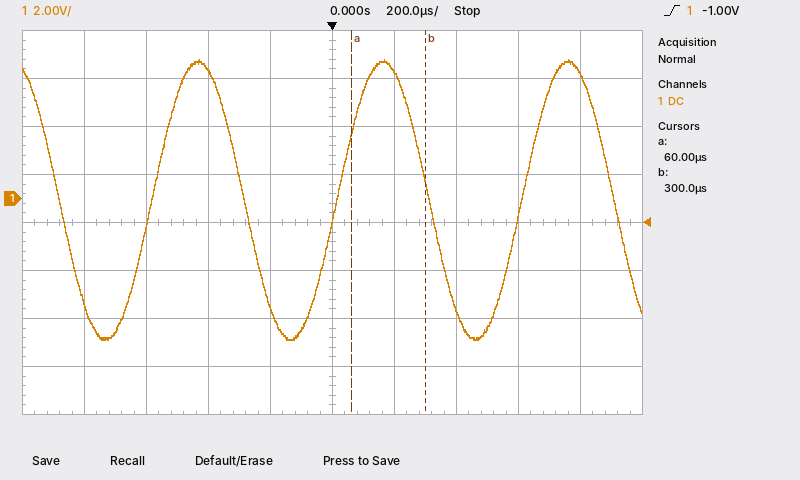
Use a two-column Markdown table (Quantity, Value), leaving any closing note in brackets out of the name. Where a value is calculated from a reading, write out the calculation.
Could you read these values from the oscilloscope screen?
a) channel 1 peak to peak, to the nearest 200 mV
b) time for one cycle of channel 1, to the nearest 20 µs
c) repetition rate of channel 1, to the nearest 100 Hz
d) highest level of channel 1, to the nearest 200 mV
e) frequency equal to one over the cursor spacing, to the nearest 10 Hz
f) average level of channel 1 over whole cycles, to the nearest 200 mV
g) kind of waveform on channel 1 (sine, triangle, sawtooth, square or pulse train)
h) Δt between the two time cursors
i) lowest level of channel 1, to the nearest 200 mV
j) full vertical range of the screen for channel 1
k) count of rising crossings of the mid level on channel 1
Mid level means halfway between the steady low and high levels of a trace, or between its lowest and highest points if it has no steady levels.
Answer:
| Quantity | Value |
|---|---|
| channel 1 peak to peak, to the nearest 200 mV | 5.8 V − (-5.8 V) = 11.6 V |
| time for one cycle of channel 1, to the nearest 20 µs | 600 µs |
| repetition rate of channel 1, to the nearest 100 Hz | 1 / 600 µs ≈ 1.7 kHz |
| highest level of channel 1, to the nearest 200 mV | 5.8 V |
| frequency equal to one over the cursor spacing, to the nearest 10 Hz | 1 / 240 µs ≈ 4.17 kHz |
| average level of channel 1 over whole cycles, to the nearest 200 mV | (5.8 V + (-5.8 V)) / 2 ≈ 0.0 V |
| kind of waveform on channel 1 | sine |
| Δt between the two time cursors | 300 µs − (60 µs) = 240 µs |
| lowest level of channel 1, to the nearest 200 mV | -5.8 V |
| full vertical range of the screen for channel 1 | 16 V |
| count of rising crossings of the mid level on channel 1 | 3 |
